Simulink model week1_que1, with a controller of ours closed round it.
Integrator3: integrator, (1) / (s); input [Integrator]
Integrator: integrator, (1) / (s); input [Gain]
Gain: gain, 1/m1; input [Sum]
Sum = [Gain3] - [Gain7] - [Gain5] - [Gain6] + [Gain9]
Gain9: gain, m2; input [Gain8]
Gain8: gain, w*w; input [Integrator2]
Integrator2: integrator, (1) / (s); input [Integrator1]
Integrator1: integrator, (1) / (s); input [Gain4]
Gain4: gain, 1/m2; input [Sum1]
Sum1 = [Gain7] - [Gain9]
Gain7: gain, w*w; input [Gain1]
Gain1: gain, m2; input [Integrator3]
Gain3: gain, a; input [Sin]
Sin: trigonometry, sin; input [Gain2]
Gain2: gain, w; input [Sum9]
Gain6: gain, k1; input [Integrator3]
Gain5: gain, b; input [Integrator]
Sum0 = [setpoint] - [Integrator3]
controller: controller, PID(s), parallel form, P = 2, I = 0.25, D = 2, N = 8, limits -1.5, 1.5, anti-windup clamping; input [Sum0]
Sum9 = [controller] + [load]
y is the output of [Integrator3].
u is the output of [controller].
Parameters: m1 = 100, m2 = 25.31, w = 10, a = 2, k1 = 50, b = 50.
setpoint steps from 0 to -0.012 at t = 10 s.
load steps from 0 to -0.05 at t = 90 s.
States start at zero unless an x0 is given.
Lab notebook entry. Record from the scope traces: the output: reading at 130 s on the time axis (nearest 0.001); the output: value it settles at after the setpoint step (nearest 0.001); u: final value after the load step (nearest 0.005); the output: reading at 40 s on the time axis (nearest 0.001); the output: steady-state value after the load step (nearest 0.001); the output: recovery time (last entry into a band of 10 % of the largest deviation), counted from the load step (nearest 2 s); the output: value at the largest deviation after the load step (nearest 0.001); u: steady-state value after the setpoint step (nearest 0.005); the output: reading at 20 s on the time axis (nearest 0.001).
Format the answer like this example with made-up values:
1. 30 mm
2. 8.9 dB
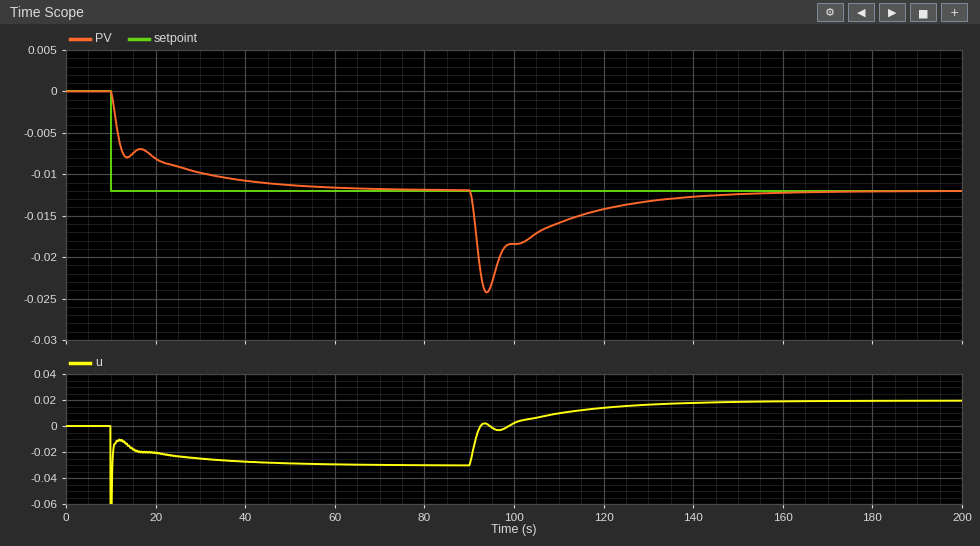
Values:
1. -0.013
2. -0.012
3. 0.020
4. -0.011
5. -0.012
6. 40 s
7. -0.024
8. -0.030
9. -0.008
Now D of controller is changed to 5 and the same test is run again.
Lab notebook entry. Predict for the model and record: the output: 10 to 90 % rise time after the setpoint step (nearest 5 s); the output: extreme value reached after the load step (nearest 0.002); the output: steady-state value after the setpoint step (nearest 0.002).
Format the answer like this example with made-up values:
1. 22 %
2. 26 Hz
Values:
1. 30 s
2. -0.022
3. -0.012
